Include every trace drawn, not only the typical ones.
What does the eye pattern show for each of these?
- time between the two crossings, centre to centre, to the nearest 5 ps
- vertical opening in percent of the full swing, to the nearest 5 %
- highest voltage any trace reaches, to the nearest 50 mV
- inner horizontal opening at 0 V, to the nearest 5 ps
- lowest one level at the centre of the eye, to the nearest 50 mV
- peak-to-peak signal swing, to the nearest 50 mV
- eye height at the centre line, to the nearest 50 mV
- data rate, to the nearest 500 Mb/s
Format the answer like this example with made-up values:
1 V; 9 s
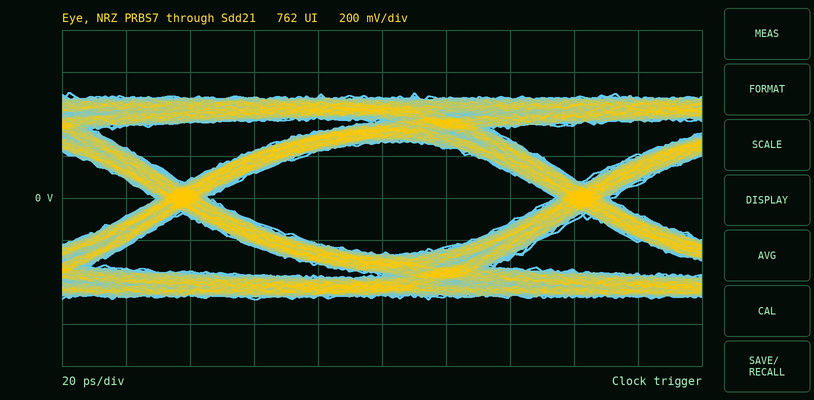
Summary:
125 ps; 55 %; 500 mV; 110 ps; 250 mV; 1.00 V; 550 mV; 8.0 Gb/s
